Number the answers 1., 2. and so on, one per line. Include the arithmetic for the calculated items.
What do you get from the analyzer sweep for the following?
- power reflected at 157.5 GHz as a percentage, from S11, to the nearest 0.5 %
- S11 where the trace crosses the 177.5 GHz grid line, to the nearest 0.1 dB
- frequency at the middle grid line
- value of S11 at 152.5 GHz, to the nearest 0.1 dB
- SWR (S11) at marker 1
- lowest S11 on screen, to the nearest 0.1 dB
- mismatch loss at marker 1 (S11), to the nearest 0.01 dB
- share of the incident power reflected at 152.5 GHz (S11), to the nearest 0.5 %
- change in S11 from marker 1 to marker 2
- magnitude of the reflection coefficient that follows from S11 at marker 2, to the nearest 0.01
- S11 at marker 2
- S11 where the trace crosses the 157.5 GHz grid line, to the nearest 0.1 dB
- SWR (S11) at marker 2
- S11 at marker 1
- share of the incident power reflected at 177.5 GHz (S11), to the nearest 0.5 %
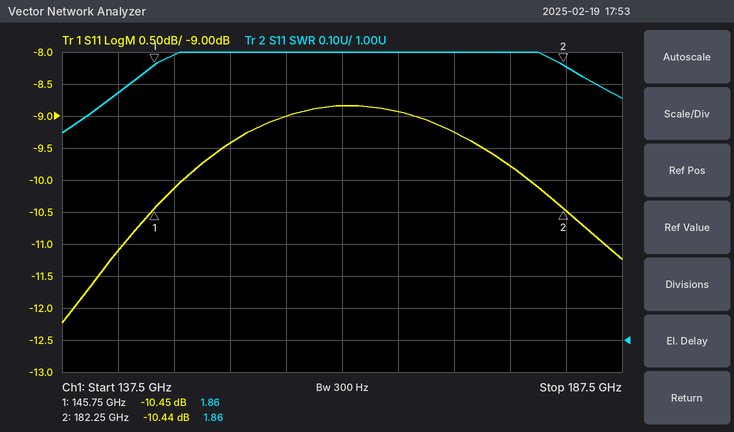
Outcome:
1. 10^(-9/10) ≈ 12.6 %, so 12.5 % to the nearest 0.5 %
2. -9.8 dB
3. 162.5 GHz
4. -9.4 dB
5. 1.86
6. -12.2 dB
7. −10 log10(1 − 10^(-10.45/10)) ≈ 0.41 dB
8. 10^(-9.4/10) ≈ 11.5 %
9. -10.44 − (-10.45) = 0.01 dB
10. 10^(-10.44/20) ≈ 0.30
11. -10.44 dB
12. -9.0 dB
13. 1.86
14. -10.45 dB
15. 10^(-9.8/10) ≈ 10.5 %
